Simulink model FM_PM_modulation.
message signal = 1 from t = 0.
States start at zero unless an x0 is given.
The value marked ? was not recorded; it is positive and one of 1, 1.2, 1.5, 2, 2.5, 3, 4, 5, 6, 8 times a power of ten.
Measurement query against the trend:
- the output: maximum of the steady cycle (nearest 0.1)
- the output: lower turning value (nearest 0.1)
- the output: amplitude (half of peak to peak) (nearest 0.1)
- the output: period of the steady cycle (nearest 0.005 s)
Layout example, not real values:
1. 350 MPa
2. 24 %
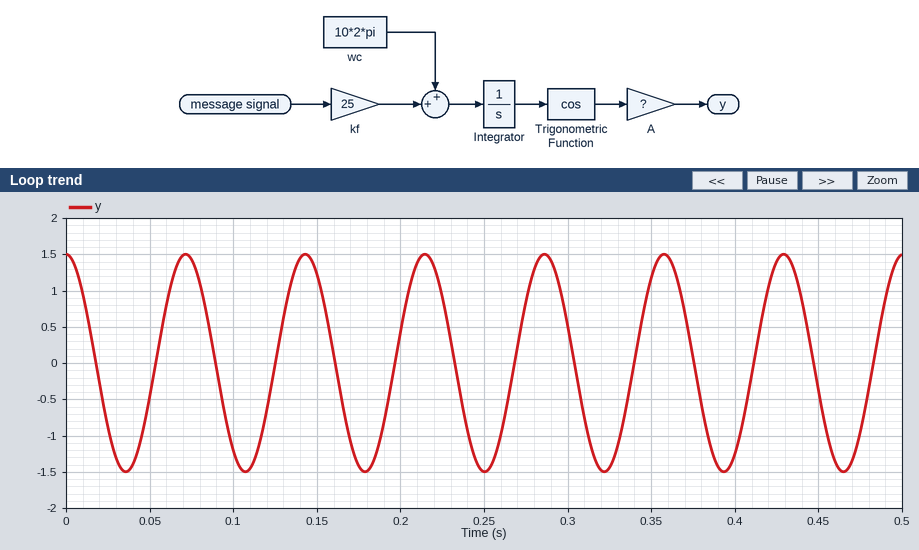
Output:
1. 1.5
2. -1.5
3. 1.5
4. 0.070 s
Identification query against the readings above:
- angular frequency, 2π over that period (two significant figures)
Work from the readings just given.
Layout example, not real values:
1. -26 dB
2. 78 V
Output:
1. 90 rad/s
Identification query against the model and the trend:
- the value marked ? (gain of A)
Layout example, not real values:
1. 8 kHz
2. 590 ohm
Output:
1. 1.5
